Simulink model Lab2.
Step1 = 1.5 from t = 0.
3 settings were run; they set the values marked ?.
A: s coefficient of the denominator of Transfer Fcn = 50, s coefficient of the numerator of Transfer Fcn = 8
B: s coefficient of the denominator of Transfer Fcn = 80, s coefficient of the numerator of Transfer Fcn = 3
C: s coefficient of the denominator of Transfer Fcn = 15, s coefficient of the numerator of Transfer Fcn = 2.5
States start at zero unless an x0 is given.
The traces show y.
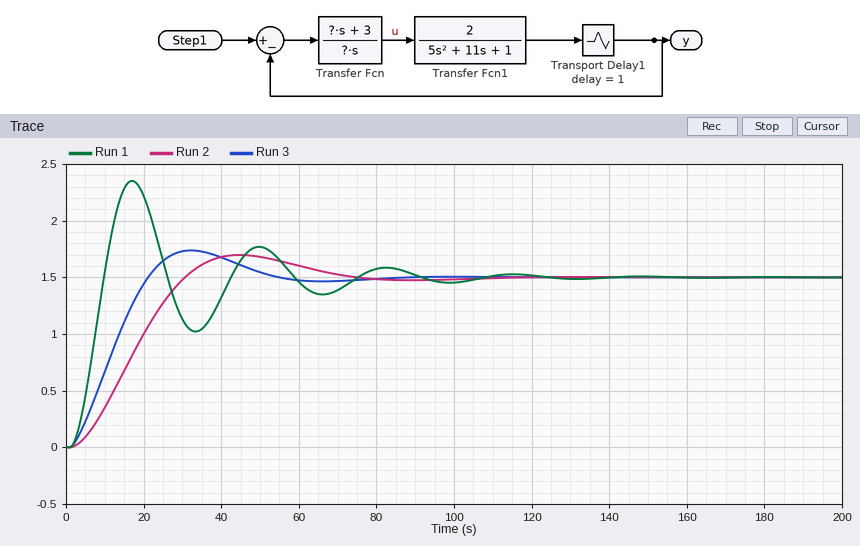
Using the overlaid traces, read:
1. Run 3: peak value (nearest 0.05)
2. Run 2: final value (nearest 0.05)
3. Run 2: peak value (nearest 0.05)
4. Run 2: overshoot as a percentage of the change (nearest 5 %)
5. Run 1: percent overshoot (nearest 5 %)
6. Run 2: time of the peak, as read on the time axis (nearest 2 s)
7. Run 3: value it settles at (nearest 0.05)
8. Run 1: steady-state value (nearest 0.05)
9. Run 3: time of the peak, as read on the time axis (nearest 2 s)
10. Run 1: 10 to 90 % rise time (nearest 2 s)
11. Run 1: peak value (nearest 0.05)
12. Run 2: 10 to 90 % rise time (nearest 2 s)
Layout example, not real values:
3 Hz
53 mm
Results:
1.75
1.50
1.70
15 %
55 %
44 s
1.50
1.50
32 s
6 s
2.35
20 s
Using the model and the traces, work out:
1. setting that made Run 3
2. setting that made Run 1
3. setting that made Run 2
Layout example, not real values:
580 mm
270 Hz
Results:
A
C
B
